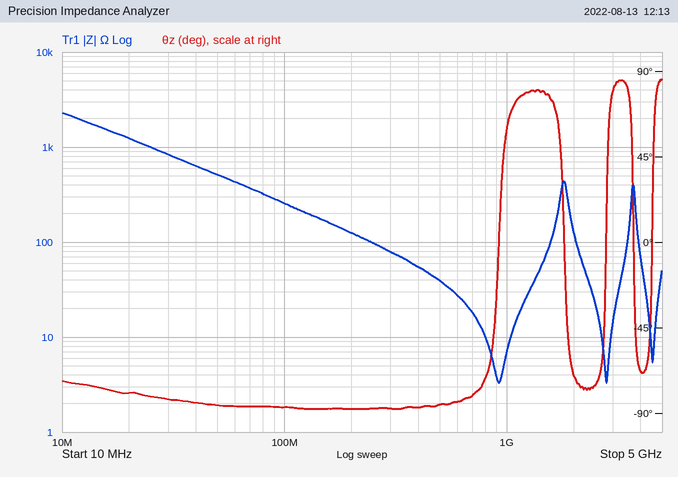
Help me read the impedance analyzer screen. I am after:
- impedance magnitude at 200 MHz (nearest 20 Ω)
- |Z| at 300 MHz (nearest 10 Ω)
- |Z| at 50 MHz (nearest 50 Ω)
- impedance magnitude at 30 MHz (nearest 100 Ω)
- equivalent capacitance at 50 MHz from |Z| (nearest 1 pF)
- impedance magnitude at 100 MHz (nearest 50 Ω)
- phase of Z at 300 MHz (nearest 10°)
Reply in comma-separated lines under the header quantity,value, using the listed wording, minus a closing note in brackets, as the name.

quantity,value
impedance magnitude at 200 MHz,120 Ω
|Z| at 300 MHz,80 Ω
|Z| at 50 MHz,500 Ω
impedance magnitude at 30 MHz,800 Ω
equivalent capacitance at 50 MHz from |Z|,6 pF
impedance magnitude at 100 MHz,250 Ω
phase of Z at 300 MHz,-90°
